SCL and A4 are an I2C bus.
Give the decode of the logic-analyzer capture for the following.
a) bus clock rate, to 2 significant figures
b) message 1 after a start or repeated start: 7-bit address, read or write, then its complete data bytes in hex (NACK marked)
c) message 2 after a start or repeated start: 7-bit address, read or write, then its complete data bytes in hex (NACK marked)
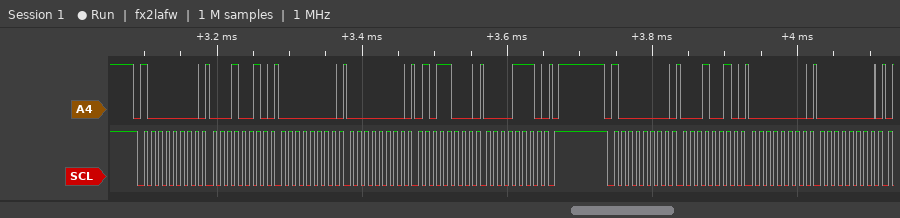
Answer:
100 kHz
0x40 write: 12 00 00 58 0E
0x40 write: 12 00 00
